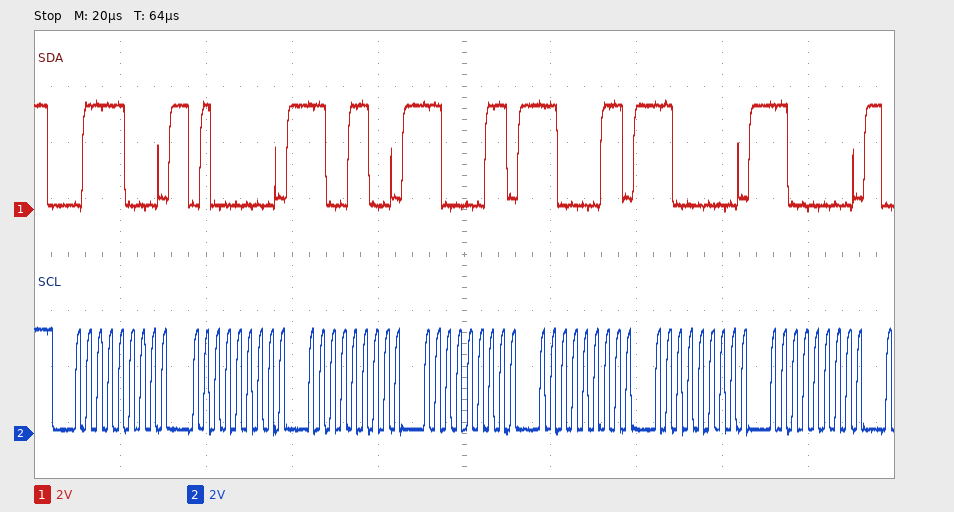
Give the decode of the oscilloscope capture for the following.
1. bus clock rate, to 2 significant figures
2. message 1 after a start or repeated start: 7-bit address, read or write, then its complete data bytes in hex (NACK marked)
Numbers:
400 kHz
0x3C write: 40 CC C3 C3 C0 C0
